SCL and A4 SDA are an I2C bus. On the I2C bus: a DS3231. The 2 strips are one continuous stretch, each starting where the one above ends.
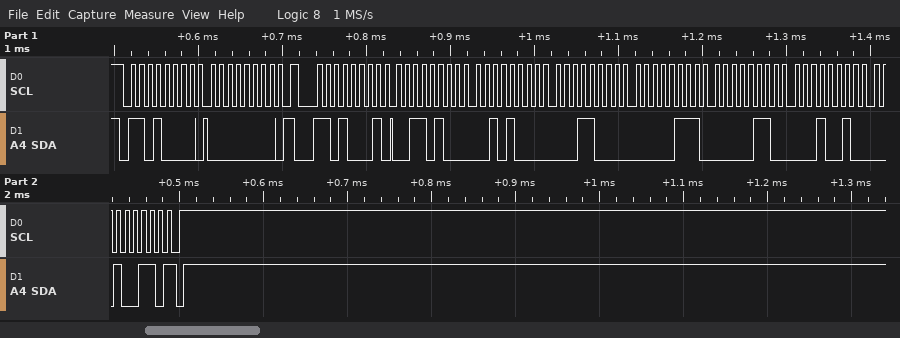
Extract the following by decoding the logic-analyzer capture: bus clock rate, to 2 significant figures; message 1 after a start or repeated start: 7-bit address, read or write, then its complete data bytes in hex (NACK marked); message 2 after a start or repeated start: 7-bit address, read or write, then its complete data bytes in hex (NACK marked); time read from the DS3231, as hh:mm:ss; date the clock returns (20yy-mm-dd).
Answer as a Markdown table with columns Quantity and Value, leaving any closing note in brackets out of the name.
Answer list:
| Quantity | Value |
|---|---|
| bus clock rate, to 2 significant figures | 100 kHz |
| message 1 after a start or repeated start: 7-bit address, read or write, then its complete data bytes in hex | 0x68 write: 00 |
| message 2 after a start or repeated start: 7-bit address, read or write, then its complete data bytes in hex | 0x68 read: 34 28 18 07 06 12 26 NACK |
| time read from the DS3231, as hh:mm:ss | 18:28:34 |
| date the clock returns | 2026-12-06 |
